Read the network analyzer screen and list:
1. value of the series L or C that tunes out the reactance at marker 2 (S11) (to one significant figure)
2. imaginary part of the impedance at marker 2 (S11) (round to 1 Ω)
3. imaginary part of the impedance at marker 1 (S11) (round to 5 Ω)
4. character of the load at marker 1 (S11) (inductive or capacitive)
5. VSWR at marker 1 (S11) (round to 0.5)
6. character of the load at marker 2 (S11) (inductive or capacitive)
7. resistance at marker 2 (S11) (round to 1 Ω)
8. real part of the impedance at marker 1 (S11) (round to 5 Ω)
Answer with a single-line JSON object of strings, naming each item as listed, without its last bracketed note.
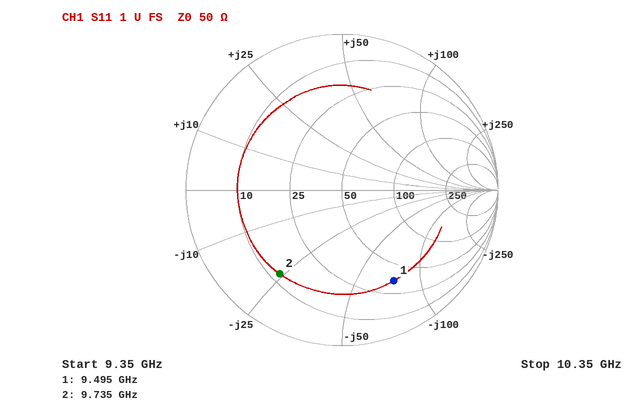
{"value of the series L or C that tunes out the reactance at marker 2 (S11)": "400 pH", "imaginary part of the impedance at marker 2 (S11)": "-24 Ω", "imaginary part of the impedance at marker 1 (S11)": "-75 Ω", "character of the load at marker 1 (S11)": "capacitive", "VSWR at marker 1 (S11)": "5.0", "character of the load at marker 2 (S11)": "capacitive", "resistance at marker 2 (S11)": "12 Ω", "real part of the impedance at marker 1 (S11)": "35 Ω"}
